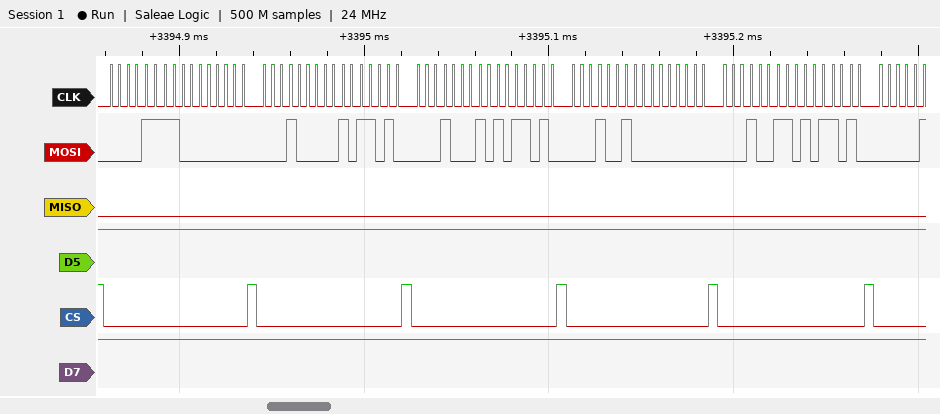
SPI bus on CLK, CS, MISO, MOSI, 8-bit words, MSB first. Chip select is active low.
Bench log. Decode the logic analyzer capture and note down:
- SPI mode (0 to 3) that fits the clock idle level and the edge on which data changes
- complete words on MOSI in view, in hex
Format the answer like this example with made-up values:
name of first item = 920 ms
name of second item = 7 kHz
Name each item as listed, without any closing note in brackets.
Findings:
SPI mode (0 to 3) that fits the clock idle level and the edge on which data changes = 0
complete words on MOSI in view, in hex = 0F, 00, 10, 5A, 11, 5A, 12, 00, 13, 5A
